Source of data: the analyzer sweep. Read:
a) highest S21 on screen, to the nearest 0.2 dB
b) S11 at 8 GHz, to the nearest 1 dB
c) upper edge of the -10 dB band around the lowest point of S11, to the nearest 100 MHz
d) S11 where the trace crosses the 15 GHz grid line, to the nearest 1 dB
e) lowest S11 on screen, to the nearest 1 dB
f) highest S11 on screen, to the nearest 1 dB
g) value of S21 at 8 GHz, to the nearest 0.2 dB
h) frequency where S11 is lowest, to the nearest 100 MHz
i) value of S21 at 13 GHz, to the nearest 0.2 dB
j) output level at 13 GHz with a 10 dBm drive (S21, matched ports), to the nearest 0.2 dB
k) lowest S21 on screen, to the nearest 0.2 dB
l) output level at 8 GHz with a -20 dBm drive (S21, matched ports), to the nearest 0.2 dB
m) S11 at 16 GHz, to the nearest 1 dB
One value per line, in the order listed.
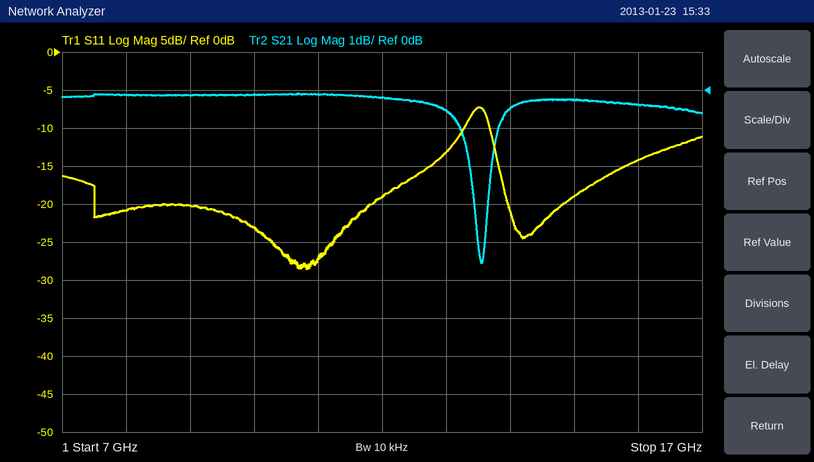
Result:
0.0 dB
-21 dB
13.3 GHz
-19 dB
-29 dB
-7 dB
-0.2 dB
10.8 GHz
-0.6 dB
9.4 dBm
-4.6 dB
-20.2 dBm
-14 dB
